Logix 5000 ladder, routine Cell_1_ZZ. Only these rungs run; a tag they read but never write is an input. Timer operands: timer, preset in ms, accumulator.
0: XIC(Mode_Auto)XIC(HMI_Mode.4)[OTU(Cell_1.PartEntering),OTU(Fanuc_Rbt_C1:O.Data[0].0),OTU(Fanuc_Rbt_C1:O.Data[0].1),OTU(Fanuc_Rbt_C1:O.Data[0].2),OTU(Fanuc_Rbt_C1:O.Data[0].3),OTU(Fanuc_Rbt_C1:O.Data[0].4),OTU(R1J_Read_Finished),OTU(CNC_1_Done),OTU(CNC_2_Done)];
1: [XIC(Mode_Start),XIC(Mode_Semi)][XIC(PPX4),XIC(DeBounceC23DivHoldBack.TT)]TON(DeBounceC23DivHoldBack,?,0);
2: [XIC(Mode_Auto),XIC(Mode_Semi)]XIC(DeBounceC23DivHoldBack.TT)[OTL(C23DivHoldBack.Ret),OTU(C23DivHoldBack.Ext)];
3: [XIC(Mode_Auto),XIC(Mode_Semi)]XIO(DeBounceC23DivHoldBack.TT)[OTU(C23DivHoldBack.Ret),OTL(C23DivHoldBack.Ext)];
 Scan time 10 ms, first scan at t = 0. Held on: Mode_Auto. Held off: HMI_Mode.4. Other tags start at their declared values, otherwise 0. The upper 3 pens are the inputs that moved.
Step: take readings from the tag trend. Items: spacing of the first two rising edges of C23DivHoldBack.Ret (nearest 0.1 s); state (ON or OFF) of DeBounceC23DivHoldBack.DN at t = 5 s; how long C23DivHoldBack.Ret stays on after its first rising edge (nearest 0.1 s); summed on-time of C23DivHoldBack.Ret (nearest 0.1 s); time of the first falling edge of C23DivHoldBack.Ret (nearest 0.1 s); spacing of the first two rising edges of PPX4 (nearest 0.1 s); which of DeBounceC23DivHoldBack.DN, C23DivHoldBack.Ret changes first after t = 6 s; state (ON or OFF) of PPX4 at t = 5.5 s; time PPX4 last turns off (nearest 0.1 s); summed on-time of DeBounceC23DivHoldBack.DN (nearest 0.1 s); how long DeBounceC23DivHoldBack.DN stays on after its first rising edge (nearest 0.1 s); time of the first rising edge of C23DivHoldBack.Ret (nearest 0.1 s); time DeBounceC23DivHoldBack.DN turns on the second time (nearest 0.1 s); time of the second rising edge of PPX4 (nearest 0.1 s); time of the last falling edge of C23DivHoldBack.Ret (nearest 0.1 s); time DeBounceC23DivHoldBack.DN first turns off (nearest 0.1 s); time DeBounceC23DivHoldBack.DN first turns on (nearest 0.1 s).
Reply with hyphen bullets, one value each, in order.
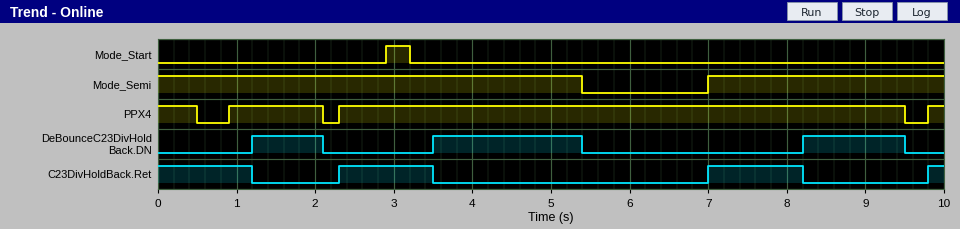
- 4.7 s
- ON
- 1.2 s
- 3.8 s
- 1.2 s
- 1.4 s
- C23DivHoldBack.Ret
- ON
- 9.5 s
- 4.1 s
- 0.9 s
- 2.3 s
- 3.5 s
- 2.3 s
- 8.2 s
- 2.1 s
- 1.2 s
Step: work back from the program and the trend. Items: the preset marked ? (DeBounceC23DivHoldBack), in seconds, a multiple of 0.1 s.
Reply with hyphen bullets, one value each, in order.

- 1.2 s
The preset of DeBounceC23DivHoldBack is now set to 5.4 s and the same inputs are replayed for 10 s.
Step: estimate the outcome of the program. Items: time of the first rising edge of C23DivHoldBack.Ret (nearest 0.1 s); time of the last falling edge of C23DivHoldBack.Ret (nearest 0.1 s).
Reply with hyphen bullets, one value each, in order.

- 7.0 s
- 5.4 s
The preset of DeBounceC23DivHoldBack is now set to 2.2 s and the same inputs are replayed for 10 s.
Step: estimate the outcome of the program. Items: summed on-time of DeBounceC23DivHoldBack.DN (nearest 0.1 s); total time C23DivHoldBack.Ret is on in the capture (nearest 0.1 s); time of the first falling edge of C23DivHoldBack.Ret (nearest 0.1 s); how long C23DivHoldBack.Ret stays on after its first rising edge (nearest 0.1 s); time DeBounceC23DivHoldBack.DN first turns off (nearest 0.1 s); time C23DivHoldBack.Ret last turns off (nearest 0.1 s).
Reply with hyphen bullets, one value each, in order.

- 1.2 s
- 6.8 s
- 2.2 s
- 2.2 s
- 2.2 s
- 9.2 s
